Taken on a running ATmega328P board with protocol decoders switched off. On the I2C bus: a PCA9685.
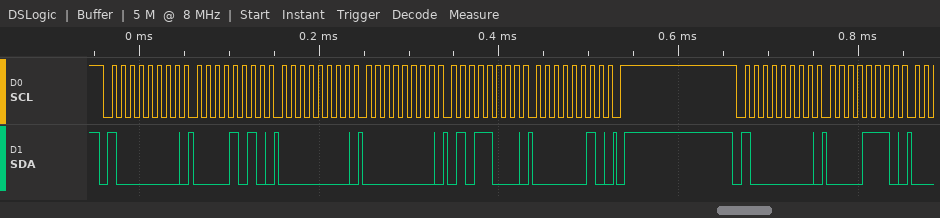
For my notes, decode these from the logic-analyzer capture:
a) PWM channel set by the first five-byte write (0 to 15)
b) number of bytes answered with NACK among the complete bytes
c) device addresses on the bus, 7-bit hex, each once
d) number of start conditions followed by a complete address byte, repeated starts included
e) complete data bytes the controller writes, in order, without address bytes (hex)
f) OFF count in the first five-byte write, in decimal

1
0
0x40
2
0A 00 00 58 02 0E
600
